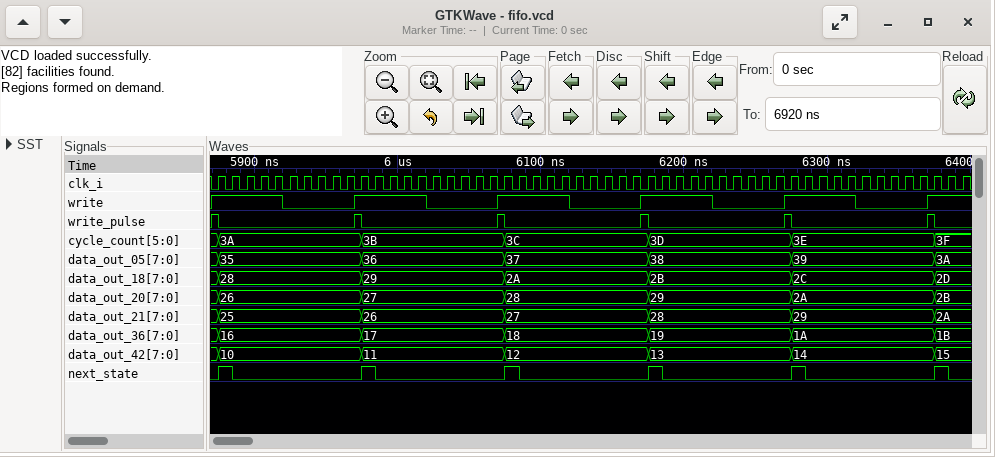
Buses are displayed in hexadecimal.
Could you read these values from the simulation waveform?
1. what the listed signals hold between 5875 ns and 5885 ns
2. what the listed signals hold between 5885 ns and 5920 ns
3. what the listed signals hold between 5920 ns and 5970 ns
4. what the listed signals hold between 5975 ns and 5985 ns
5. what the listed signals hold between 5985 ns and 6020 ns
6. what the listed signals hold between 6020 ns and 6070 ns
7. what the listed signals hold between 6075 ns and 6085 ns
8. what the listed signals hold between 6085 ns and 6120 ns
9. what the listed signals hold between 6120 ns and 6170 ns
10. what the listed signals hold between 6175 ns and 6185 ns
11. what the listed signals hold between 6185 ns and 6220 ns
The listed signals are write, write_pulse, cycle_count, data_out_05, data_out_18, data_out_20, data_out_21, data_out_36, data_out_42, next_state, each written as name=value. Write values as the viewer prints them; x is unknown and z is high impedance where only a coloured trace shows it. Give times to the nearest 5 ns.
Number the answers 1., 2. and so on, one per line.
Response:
1. write=1, write_pulse=0, cycle_count=3A, data_out_05=35, data_out_18=28, data_out_20=26, data_out_21=25, data_out_36=16, data_out_42=10, next_state=1
2. write=1, write_pulse=0, cycle_count=3A, data_out_05=35, data_out_18=28, data_out_20=26, data_out_21=25, data_out_36=16, data_out_42=10, next_state=0
3. write=0, write_pulse=0, cycle_count=3A, data_out_05=35, data_out_18=28, data_out_20=26, data_out_21=25, data_out_36=16, data_out_42=10, next_state=0
4. write=1, write_pulse=0, cycle_count=3B, data_out_05=36, data_out_18=29, data_out_20=27, data_out_21=26, data_out_36=17, data_out_42=11, next_state=1
5. write=1, write_pulse=0, cycle_count=3B, data_out_05=36, data_out_18=29, data_out_20=27, data_out_21=26, data_out_36=17, data_out_42=11, next_state=0
6. write=0, write_pulse=0, cycle_count=3B, data_out_05=36, data_out_18=29, data_out_20=27, data_out_21=26, data_out_36=17, data_out_42=11, next_state=0
7. write=1, write_pulse=0, cycle_count=3C, data_out_05=37, data_out_18=2A, data_out_20=28, data_out_21=27, data_out_36=18, data_out_42=12, next_state=1
8. write=1, write_pulse=0, cycle_count=3C, data_out_05=37, data_out_18=2A, data_out_20=28, data_out_21=27, data_out_36=18, data_out_42=12, next_state=0
9. write=0, write_pulse=0, cycle_count=3C, data_out_05=37, data_out_18=2A, data_out_20=28, data_out_21=27, data_out_36=18, data_out_42=12, next_state=0
10. write=1, write_pulse=0, cycle_count=3D, data_out_05=38, data_out_18=2B, data_out_20=29, data_out_21=28, data_out_36=19, data_out_42=13, next_state=1
11. write=1, write_pulse=0, cycle_count=3D, data_out_05=38, data_out_18=2B, data_out_20=29, data_out_21=28, data_out_36=19, data_out_42=13, next_state=0
